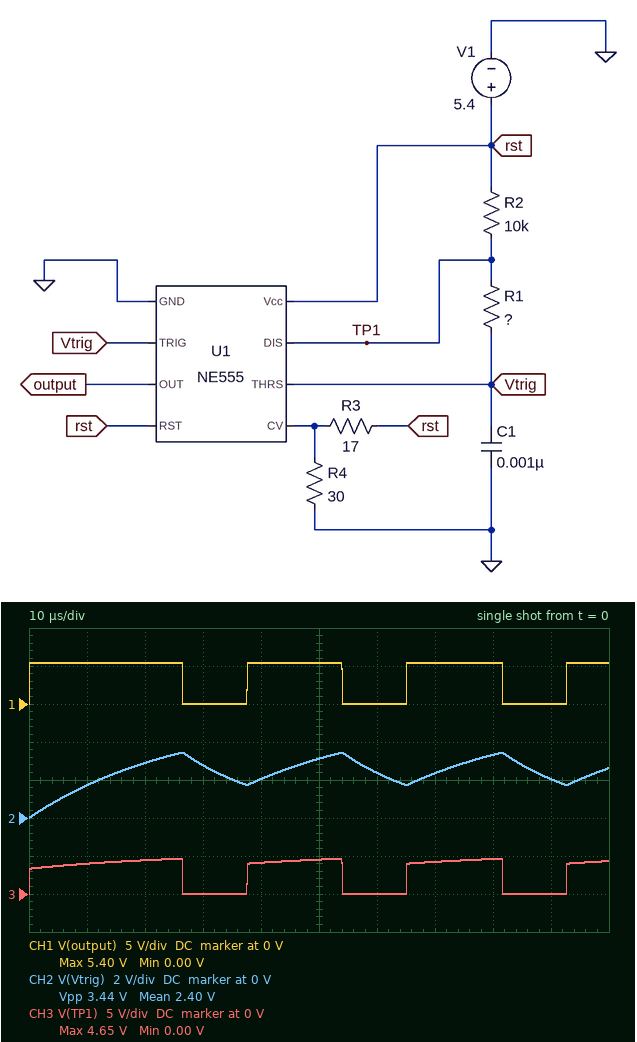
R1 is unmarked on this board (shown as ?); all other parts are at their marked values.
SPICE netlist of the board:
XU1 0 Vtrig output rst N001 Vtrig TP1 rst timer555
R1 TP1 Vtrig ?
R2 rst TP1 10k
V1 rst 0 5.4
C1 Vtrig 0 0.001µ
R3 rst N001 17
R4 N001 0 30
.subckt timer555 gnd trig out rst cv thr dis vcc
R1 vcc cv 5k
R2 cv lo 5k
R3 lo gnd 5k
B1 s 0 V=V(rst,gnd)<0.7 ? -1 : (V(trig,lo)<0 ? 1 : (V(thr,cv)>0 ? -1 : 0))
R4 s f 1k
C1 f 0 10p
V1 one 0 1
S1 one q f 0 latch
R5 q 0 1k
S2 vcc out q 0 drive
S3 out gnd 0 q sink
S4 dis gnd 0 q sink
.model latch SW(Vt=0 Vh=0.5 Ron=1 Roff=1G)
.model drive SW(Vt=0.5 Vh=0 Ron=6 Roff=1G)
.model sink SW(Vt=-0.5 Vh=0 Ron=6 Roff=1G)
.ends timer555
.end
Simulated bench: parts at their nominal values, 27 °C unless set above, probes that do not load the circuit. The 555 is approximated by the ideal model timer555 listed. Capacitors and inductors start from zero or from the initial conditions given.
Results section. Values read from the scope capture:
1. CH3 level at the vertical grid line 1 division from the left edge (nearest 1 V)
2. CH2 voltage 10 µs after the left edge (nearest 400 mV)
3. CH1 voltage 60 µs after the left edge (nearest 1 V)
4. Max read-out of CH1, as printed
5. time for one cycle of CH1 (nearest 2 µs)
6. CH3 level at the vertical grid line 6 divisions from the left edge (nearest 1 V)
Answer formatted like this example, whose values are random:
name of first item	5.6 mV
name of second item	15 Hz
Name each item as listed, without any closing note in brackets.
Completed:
CH3 level at the vertical grid line 1 division from the left edge	4 V
CH2 voltage 10 µs after the left edge	1.6 V
CH1 voltage 60 µs after the left edge	0 V
Max read-out of CH1, as printed	5.40 V
time for one cycle of CH1	28 µs
CH3 level at the vertical grid line 6 divisions from the left edge	0 V
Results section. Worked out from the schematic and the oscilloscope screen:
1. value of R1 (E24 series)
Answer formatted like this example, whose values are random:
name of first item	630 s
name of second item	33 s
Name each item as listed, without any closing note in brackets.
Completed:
value of R1	16 kΩ
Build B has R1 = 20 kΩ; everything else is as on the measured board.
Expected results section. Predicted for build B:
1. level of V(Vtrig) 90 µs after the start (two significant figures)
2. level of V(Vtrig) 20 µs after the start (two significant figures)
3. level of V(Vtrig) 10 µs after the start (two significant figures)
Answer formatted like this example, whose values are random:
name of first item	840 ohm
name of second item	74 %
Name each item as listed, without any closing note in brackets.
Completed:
level of V(Vtrig) 90 µs after the start	3.0 V
level of V(Vtrig) 20 µs after the start	2.6 V
level of V(Vtrig) 10 µs after the start	1.5 V
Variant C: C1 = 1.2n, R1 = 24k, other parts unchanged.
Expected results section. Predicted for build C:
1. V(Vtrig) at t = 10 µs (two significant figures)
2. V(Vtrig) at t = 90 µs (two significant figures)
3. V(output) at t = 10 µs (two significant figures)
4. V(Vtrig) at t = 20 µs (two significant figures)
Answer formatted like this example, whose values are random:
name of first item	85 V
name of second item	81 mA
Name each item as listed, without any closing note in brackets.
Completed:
V(Vtrig) at t = 10 µs	1.2 V
V(Vtrig) at t = 90 µs	3.1 V
V(output) at t = 10 µs	5.4 V
V(Vtrig) at t = 20 µs	2.1 V
